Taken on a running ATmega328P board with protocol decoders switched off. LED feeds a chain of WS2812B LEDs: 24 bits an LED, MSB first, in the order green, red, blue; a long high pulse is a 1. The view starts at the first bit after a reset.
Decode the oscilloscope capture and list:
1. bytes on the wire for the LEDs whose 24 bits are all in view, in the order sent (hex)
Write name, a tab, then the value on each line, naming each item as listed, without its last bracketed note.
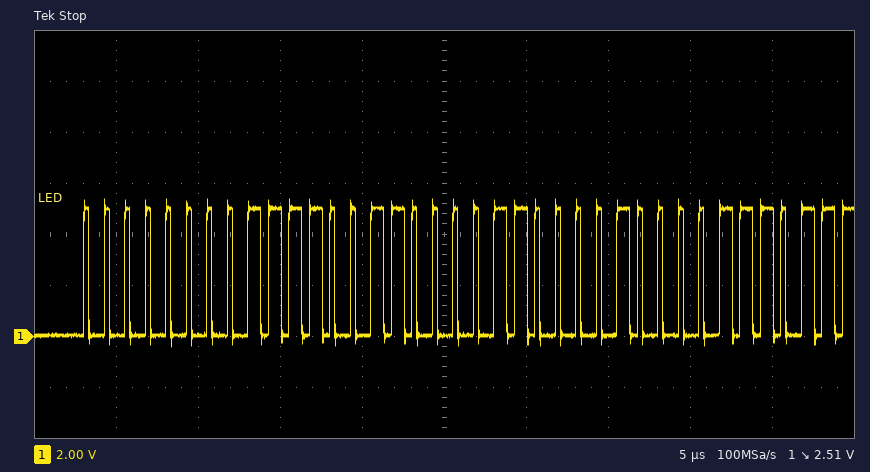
bytes on the wire for the LEDs whose 24 bits are all in view, in the order sent	00 F3 0C
